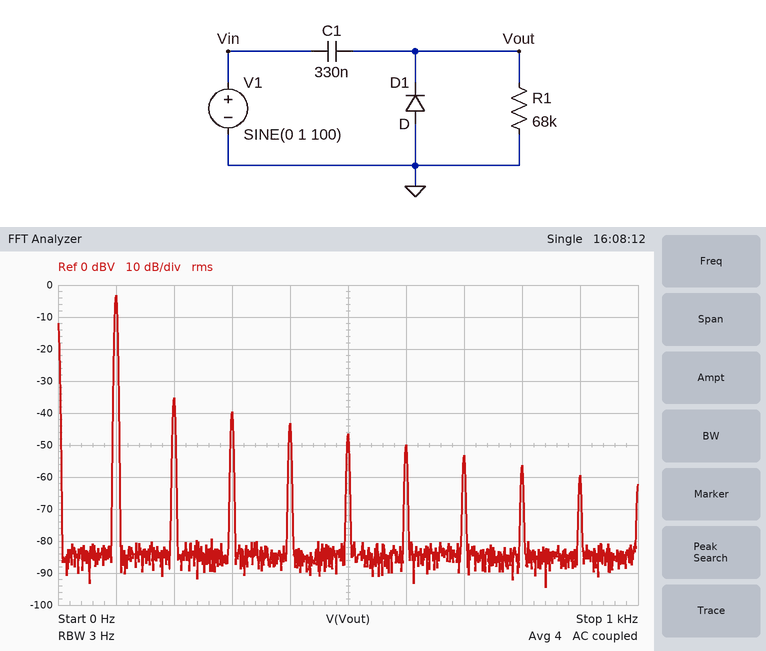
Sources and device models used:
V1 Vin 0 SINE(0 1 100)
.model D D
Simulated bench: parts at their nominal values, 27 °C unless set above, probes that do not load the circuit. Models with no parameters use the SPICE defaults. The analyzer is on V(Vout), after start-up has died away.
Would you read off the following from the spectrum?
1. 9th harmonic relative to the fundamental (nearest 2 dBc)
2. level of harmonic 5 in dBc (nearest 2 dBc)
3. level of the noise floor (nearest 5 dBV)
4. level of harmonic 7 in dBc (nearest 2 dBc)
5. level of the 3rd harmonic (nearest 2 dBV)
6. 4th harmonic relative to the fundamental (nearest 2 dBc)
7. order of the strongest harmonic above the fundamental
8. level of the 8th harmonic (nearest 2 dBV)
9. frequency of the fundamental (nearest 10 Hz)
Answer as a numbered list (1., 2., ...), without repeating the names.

1. -56 dBc
2. -44 dBc
3. -85 dBV
4. -50 dBc
5. -40 dBV
6. -40 dBc
7. 2
8. -56 dBV
9. 100 Hz
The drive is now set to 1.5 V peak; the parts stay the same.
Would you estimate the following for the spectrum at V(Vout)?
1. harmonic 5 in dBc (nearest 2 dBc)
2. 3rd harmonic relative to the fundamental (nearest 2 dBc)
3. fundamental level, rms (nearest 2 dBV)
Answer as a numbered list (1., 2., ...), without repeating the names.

1. -40 dBc
2. -34 dBc
3. 0 dBV
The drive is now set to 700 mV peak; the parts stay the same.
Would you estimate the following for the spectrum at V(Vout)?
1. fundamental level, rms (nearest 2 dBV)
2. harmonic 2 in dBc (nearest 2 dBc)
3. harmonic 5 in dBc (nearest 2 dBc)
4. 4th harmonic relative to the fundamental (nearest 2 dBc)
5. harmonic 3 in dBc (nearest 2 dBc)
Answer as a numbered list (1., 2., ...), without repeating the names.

1. -6 dBV
2. -38 dBc
3. -50 dBc
4. -46 dBc
5. -42 dBc
